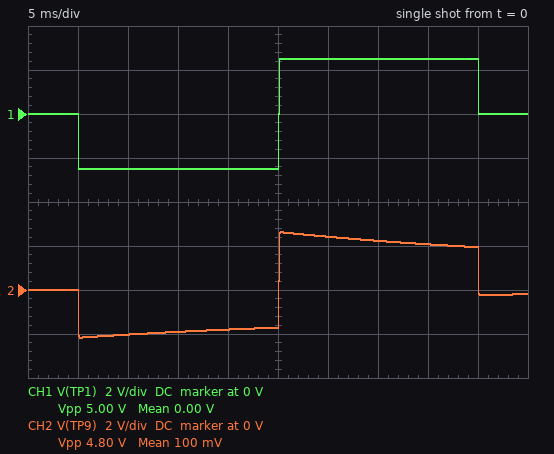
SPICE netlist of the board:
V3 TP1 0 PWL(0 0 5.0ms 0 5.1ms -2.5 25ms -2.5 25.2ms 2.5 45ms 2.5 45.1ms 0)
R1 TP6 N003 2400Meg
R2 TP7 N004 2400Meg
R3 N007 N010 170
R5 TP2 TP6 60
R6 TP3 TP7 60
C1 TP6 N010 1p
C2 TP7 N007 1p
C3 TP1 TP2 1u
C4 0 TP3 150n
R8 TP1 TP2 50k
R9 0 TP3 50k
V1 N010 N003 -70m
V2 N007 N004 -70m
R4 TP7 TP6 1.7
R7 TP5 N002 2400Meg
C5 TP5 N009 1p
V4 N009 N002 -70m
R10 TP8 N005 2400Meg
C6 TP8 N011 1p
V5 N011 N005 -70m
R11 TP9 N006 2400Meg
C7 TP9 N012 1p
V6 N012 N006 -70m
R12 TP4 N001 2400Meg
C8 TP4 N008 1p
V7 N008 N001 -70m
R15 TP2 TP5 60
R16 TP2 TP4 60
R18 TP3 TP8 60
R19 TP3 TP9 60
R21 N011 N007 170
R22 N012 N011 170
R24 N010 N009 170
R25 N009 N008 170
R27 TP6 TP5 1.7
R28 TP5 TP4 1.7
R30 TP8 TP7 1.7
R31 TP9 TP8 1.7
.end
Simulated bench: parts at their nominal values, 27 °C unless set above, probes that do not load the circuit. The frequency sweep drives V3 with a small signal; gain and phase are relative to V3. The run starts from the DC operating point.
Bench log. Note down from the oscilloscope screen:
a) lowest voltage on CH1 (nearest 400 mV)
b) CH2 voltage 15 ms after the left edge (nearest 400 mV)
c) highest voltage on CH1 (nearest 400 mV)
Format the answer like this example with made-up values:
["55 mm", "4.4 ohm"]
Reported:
["-2.4 V", "-2.0 V", "2.4 V"]
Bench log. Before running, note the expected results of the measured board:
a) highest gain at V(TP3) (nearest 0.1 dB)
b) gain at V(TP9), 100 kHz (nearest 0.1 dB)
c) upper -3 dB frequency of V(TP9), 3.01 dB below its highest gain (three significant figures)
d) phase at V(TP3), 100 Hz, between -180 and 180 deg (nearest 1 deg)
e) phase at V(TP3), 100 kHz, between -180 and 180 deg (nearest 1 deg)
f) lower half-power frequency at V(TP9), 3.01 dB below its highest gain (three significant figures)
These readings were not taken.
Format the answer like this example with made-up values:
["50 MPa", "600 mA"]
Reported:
["-1.2 dB", "-6.3 dB", "40.4 kHz", "1 deg", "-74 deg", "3.22 Hz"]
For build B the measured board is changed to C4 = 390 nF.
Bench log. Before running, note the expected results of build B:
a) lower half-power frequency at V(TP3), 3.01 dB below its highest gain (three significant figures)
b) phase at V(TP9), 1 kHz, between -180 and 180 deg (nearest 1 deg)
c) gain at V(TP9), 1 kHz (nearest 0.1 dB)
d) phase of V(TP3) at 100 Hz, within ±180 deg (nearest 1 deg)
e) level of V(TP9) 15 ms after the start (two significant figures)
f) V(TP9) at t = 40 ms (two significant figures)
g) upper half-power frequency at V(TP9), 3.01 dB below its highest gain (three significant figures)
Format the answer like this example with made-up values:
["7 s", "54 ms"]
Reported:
["835 mHz", "-2 deg", "-2.9 dB", "0 deg", "-1.7 V", "1.8 V", "26.5 kHz"]
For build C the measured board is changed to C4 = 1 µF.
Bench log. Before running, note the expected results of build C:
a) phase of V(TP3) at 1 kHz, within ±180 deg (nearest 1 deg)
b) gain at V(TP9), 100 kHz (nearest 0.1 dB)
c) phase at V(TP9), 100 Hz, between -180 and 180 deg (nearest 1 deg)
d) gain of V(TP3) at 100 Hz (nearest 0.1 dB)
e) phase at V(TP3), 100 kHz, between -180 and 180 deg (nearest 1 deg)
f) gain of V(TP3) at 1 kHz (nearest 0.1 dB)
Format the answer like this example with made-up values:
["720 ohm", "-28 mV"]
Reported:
["-8 deg", "-7.1 dB", "0 deg", "-6.0 dB", "-86 deg", "-6.1 dB"]
